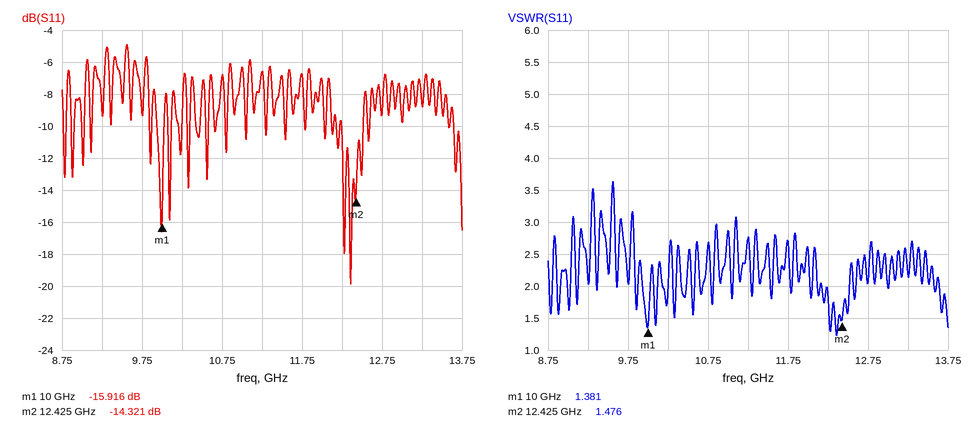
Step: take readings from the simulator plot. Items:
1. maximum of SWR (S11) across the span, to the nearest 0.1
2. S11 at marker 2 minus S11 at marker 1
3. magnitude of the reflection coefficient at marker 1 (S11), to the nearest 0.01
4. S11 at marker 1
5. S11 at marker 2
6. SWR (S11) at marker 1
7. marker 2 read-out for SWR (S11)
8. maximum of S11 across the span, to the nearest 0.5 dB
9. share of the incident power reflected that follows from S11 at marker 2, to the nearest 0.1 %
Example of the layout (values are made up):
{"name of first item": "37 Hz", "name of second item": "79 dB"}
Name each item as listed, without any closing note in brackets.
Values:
{"maximum of SWR (S11) across the span, to the nearest 0.1": "3.6", "S11 at marker 2 minus S11 at marker 1": "1.595 dB", "magnitude of the reflection coefficient at marker 1 (S11), to the nearest 0.01": "0.16", "S11 at marker 1": "-15.916 dB", "S11 at marker 2": "-14.321 dB", "SWR (S11) at marker 1": "1.381", "marker 2 read-out for SWR": "1.476", "maximum of S11 across the span, to the nearest 0.5 dB": "-5.0 dB", "share of the incident power reflected that follows from S11 at marker 2, to the nearest 0.1 %": "3.7 %"}
